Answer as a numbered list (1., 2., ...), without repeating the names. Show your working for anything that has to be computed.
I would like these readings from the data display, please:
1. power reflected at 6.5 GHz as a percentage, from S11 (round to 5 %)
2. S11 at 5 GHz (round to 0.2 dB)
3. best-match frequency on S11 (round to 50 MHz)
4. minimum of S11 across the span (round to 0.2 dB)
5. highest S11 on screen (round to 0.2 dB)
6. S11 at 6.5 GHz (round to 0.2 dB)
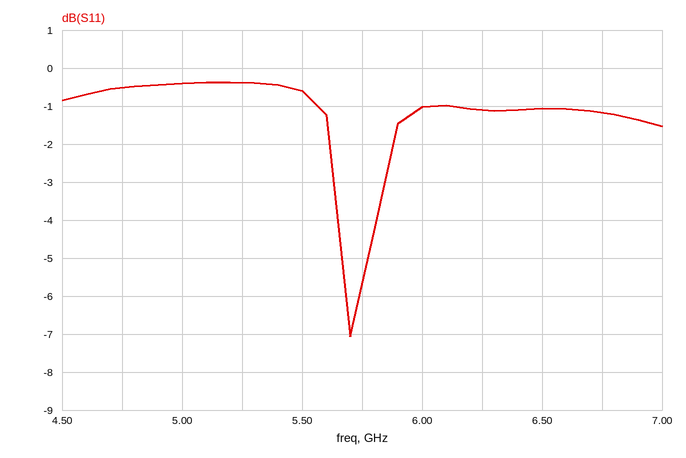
1. 10^(-1/10) ≈ 79.4 %, so 80 % to the nearest 5 %
2. -0.4 dB
3. 5.70 GHz
4. -7.0 dB
5. -0.4 dB
6. -1.0 dB
